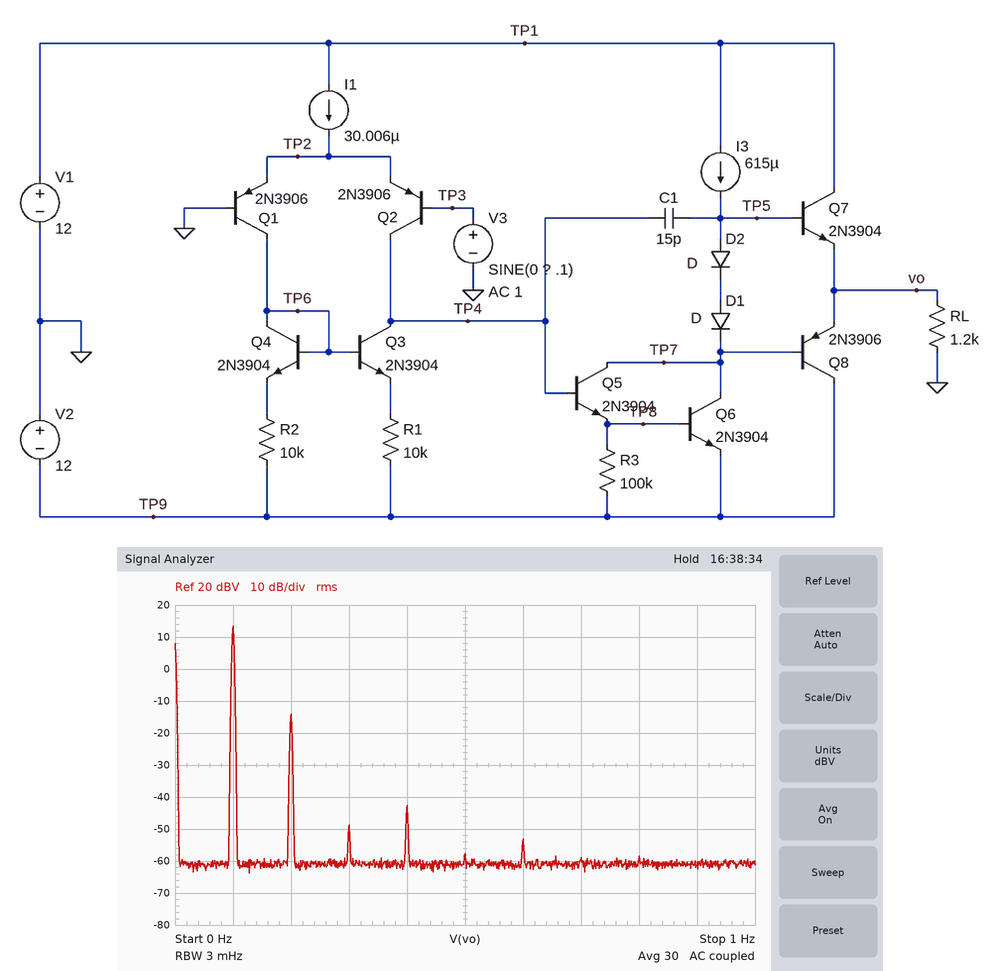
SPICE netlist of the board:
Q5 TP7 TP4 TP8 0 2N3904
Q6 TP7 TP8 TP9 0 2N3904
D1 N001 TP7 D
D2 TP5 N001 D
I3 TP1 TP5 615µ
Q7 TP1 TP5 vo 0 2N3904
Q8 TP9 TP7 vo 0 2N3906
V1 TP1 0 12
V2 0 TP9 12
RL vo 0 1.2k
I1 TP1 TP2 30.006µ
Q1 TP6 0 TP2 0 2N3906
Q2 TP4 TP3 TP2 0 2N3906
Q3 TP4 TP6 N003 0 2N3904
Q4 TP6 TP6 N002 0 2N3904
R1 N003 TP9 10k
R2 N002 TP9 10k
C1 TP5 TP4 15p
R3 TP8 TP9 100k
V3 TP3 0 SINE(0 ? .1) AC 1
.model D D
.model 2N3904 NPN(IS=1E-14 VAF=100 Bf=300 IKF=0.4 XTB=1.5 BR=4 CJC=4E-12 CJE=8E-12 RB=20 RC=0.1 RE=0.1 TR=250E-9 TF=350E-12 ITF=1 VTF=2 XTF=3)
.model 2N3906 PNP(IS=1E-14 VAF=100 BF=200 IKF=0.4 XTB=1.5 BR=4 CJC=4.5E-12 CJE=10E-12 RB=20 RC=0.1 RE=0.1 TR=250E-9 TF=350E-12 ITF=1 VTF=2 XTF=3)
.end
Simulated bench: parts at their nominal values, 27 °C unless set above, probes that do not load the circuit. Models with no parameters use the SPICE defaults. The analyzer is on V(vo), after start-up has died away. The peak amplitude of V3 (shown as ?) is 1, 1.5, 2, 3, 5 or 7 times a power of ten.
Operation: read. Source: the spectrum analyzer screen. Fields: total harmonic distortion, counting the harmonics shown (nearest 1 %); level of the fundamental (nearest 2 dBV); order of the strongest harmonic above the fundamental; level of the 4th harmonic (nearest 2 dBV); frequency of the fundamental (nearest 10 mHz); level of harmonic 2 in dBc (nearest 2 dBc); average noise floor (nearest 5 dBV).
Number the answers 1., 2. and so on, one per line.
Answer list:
1. 4 %
2. 14 dBV
3. 2
4. -42 dBV
5. 100 mHz
6. -28 dBc
7. -60 dBV
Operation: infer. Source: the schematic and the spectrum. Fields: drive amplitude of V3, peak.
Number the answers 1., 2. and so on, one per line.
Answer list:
1. 5 µV
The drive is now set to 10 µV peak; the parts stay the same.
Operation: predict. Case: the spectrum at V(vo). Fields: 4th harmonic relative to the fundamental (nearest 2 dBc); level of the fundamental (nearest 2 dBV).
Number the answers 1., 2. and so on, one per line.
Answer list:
1. -32 dBc
2. 18 dBV
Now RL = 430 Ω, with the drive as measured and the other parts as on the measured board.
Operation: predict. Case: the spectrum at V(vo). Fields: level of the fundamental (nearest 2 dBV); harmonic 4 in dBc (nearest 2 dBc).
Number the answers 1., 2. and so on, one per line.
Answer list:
1. 12 dBV
2. -46 dBc
